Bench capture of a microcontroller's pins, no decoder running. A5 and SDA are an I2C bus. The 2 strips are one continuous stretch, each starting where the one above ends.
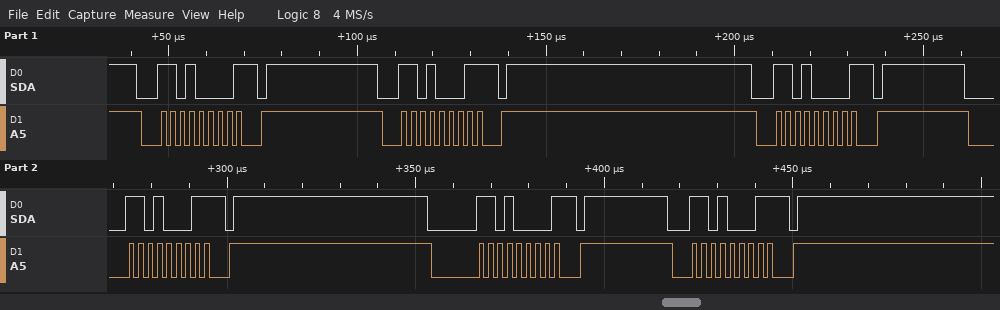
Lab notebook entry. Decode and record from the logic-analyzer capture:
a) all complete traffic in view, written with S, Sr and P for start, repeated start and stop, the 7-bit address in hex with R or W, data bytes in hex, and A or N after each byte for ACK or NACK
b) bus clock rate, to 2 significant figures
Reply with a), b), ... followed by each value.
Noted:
a) S 68W N P S 68R N P S 68W N P S 68R N P S 68W N P S 68R N P
b) 400 kHz
